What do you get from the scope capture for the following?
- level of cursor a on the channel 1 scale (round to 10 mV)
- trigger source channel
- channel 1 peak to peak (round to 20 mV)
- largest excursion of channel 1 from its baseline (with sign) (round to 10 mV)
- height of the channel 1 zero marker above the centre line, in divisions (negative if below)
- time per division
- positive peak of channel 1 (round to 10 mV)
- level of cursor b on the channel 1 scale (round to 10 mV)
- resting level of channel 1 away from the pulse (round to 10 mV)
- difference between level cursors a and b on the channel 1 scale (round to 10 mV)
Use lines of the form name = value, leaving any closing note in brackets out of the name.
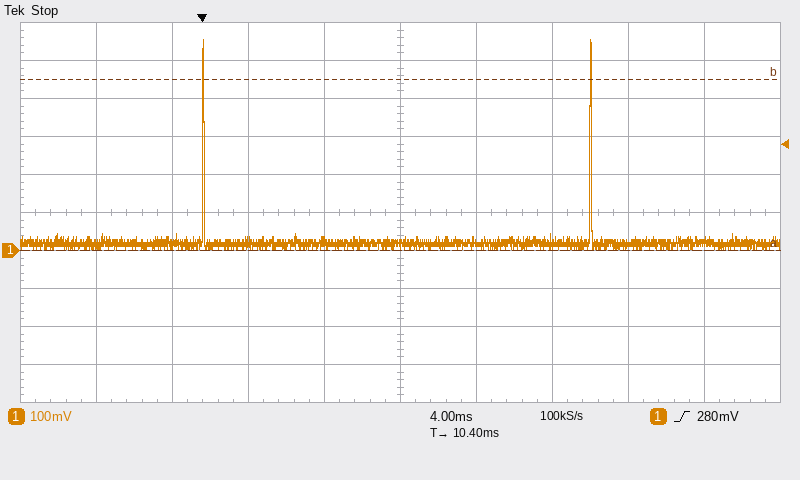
level of cursor a on the channel 1 scale = 0 mV
trigger source channel = channel 1
channel 1 peak to peak = 560 mV
largest excursion of channel 1 from its baseline (with sign) = +540 mV
height of the channel 1 zero marker above the centre line, in divisions = -1.0 div
time per division = 4 ms
positive peak of channel 1 = 560 mV
level of cursor b on the channel 1 scale = 450 mV
resting level of channel 1 away from the pulse = 20 mV
difference between level cursors a and b on the channel 1 scale = 450 mV
